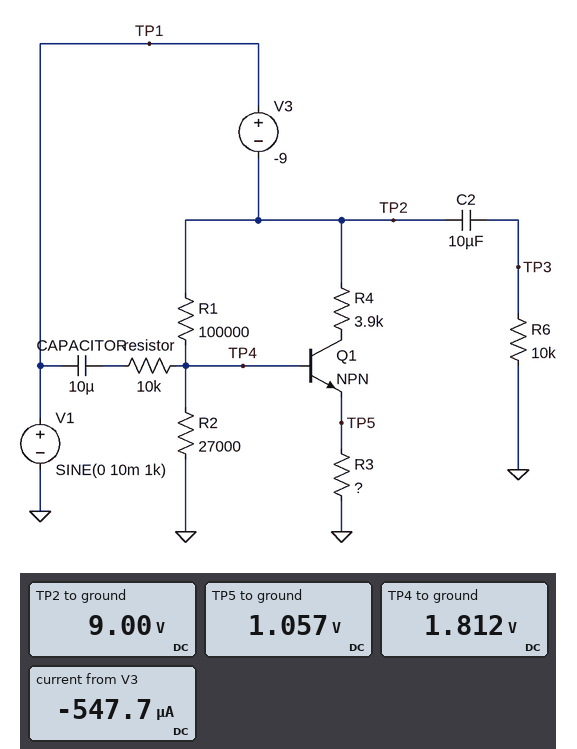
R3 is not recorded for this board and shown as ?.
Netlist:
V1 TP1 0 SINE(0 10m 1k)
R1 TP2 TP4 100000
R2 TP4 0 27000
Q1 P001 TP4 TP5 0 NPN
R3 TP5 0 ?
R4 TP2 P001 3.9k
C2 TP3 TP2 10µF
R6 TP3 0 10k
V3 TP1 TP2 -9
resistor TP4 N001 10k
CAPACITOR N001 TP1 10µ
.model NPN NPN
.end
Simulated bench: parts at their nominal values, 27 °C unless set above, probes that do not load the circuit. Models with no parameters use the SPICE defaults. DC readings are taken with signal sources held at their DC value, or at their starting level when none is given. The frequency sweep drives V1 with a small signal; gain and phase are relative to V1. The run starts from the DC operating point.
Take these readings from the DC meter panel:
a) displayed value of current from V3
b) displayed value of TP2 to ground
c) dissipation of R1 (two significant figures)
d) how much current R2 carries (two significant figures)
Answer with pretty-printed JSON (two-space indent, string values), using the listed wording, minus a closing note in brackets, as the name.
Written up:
{
  "displayed value of current from V3": "-547.7 µA",
  "displayed value of TP2 to ground": "9.00 V",
  "dissipation of R1": "520 µW",
  "how much current R2 carries": "67 µA"
}
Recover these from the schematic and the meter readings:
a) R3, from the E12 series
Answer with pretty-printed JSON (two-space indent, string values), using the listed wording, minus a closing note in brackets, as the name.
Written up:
{
  "R3, from the E12 series": "2.2 kΩ"
}
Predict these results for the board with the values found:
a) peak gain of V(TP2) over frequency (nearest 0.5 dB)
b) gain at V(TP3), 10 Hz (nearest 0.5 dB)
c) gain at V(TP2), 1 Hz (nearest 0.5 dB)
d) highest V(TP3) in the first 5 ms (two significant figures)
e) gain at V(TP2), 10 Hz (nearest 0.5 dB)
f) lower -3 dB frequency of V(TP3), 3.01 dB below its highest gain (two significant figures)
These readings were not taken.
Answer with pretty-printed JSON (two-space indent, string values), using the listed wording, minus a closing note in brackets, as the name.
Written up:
{
  "peak gain of V(TP2) over frequency": "0 dB",
  "gain at V(TP3), 10 Hz": "0 dB",
  "gain at V(TP2), 1 Hz": "0 dB",
  "highest V(TP3) in the first 5 ms": "10 mV",
  "gain at V(TP2), 10 Hz": "0 dB",
  "lower -3 dB frequency of V(TP3), 3.01 dB below its highest gain": "1.6 Hz"
}
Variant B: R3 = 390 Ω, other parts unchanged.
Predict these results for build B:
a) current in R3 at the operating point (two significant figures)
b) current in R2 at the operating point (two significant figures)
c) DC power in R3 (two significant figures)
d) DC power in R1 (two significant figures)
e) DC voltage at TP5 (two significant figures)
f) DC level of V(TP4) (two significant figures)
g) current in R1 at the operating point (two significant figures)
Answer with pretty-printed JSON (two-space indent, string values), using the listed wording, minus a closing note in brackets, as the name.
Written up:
{
  "current in R3 at the operating point": "1.9 mA",
  "current in R2 at the operating point": "56 µA",
  "DC power in R3": "1.4 mW",
  "DC power in R1": "560 µW",
  "DC voltage at TP5": "730 mV",
  "DC level of V(TP4)": "1.5 V",
  "current in R1 at the operating point": "75 µA"
}
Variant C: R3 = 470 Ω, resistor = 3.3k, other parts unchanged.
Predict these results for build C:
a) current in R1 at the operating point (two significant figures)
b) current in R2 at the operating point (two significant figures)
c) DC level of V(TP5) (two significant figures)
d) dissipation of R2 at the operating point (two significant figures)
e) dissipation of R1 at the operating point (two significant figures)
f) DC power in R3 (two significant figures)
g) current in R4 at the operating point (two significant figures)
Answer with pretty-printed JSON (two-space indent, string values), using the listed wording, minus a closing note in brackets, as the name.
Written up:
{
  "current in R1 at the operating point": "74 µA",
  "current in R2 at the operating point": "58 µA",
  "DC level of V(TP5)": "780 mV",
  "dissipation of R2 at the operating point": "91 µW",
  "dissipation of R1 at the operating point": "550 µW",
  "DC power in R3": "1.3 mW",
  "current in R4 at the operating point": "1.6 mA"
}
